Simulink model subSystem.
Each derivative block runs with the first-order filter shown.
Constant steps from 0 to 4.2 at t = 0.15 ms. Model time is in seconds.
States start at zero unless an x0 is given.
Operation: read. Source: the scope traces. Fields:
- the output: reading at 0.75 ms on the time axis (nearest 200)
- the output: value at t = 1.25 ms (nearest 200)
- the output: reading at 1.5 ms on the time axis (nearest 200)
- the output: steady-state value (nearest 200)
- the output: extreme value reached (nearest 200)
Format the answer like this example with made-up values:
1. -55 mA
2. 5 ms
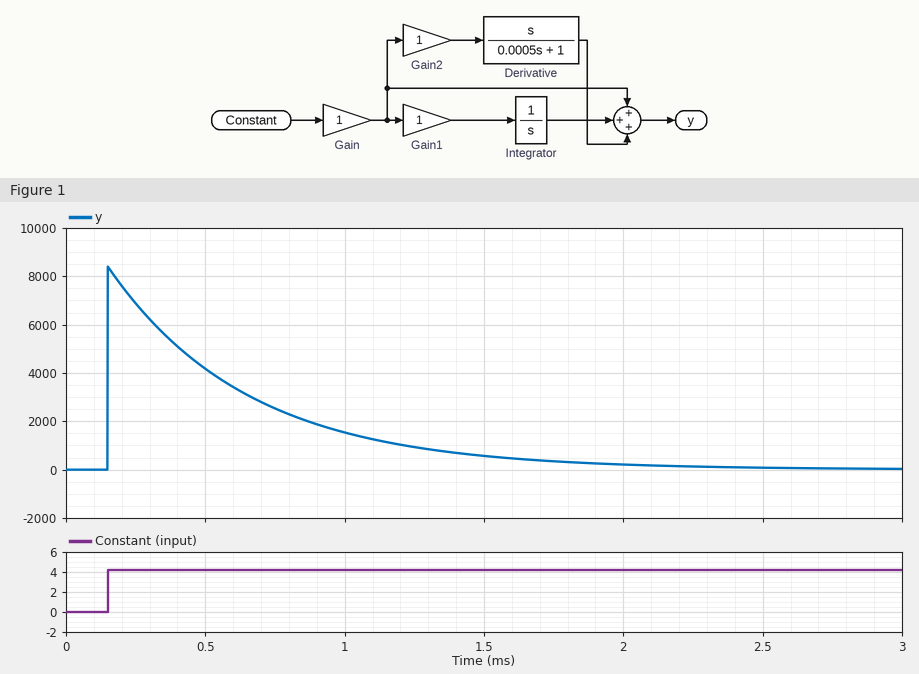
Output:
1. 2600
2. 1000
3. 600
4. 0
5. 8400
